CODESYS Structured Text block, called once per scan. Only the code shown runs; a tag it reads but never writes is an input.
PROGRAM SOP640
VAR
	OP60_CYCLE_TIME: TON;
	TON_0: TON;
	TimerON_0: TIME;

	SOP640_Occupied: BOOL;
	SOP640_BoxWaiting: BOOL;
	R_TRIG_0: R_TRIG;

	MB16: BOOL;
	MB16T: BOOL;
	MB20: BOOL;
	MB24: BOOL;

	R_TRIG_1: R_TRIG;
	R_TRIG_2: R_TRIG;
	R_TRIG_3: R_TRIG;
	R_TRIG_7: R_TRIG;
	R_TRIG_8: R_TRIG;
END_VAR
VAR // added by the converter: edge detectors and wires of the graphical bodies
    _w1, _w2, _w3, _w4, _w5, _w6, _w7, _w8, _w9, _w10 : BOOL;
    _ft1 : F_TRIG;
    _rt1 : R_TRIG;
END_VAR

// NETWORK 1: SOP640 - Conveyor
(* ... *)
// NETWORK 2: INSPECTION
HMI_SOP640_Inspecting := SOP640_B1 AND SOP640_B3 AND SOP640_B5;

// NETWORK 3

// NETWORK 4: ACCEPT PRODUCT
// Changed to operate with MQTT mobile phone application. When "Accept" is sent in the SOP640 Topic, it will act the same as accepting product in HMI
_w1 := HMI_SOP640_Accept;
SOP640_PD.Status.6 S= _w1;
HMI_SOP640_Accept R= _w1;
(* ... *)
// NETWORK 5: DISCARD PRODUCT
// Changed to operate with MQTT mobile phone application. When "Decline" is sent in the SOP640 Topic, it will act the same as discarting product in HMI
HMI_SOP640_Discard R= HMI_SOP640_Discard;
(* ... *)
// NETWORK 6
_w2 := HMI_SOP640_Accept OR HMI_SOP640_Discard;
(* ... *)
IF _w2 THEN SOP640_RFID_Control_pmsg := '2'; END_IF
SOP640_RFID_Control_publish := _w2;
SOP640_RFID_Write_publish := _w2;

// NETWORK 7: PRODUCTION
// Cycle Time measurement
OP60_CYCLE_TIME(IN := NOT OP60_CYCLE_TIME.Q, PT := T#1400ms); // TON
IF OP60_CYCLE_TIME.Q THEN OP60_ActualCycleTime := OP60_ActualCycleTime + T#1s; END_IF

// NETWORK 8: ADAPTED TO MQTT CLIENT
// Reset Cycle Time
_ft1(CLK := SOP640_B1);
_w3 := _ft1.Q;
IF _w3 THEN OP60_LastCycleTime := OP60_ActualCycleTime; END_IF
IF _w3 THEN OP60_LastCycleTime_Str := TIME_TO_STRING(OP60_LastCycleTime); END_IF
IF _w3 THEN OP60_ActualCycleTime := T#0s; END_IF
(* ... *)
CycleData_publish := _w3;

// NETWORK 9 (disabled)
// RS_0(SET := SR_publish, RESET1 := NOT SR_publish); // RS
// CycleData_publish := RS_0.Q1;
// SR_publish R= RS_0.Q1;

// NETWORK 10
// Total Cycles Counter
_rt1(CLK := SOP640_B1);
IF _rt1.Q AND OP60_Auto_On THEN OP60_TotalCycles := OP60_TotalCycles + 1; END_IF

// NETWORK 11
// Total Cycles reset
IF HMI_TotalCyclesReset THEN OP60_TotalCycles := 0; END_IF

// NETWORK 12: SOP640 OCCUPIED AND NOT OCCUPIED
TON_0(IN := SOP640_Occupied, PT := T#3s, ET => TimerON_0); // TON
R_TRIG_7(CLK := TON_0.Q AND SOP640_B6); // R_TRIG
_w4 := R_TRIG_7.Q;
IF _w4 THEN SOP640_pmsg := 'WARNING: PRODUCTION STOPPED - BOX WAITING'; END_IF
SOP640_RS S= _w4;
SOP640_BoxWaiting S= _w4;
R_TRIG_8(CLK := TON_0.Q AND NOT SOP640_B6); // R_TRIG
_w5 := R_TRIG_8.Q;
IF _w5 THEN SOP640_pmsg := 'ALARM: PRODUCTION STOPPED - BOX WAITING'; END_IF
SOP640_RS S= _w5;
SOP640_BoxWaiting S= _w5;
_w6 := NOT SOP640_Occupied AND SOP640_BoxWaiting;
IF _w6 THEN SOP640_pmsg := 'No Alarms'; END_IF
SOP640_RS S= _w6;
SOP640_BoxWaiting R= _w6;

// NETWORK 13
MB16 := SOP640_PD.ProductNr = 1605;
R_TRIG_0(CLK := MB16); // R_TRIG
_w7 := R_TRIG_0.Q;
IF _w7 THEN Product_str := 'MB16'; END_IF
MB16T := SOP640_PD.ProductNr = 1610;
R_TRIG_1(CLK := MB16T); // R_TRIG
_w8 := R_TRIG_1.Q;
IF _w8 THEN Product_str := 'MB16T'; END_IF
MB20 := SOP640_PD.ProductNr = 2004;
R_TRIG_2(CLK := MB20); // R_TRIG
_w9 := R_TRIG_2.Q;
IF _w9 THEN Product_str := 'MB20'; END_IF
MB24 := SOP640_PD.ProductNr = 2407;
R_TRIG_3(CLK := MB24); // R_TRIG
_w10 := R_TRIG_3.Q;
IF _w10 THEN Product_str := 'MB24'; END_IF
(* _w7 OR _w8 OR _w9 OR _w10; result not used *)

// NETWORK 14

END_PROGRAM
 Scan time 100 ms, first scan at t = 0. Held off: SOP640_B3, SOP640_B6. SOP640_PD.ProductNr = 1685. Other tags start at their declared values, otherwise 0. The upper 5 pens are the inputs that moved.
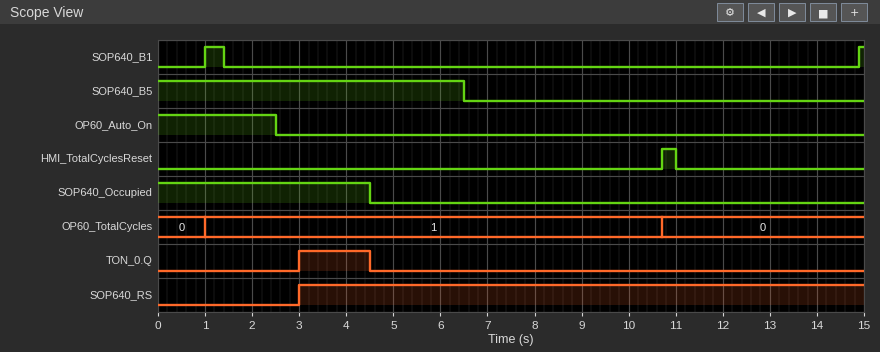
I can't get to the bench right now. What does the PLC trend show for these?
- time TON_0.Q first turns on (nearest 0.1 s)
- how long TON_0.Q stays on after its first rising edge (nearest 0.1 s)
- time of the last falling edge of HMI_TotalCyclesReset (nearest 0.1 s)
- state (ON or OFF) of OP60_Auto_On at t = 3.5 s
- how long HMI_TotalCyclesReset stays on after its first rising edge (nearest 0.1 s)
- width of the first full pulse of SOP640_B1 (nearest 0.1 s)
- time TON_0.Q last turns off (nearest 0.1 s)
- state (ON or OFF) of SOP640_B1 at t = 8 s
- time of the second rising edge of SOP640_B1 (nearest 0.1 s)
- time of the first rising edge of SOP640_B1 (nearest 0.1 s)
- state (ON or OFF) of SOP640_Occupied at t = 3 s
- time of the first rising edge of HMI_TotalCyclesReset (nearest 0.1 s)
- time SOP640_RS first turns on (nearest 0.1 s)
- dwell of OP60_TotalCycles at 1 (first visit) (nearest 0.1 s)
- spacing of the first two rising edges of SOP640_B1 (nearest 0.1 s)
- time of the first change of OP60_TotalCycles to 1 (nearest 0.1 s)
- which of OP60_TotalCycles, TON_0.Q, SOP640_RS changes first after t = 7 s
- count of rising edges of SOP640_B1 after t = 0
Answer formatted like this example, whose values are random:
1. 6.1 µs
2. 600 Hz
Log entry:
1. 3.0 s
2. 1.5 s
3. 11.0 s
4. OFF
5. 0.3 s
6. 0.4 s
7. 4.5 s
8. OFF
9. 14.9 s
10. 1.0 s
11. ON
12. 10.7 s
13. 3.0 s
14. 9.7 s
15. 13.9 s
16. 1.0 s
17. OP60_TotalCycles
18. 2
